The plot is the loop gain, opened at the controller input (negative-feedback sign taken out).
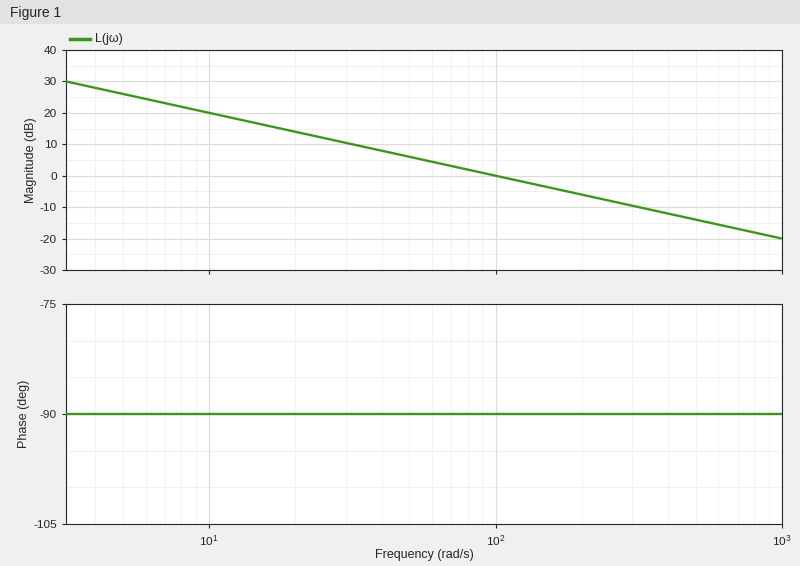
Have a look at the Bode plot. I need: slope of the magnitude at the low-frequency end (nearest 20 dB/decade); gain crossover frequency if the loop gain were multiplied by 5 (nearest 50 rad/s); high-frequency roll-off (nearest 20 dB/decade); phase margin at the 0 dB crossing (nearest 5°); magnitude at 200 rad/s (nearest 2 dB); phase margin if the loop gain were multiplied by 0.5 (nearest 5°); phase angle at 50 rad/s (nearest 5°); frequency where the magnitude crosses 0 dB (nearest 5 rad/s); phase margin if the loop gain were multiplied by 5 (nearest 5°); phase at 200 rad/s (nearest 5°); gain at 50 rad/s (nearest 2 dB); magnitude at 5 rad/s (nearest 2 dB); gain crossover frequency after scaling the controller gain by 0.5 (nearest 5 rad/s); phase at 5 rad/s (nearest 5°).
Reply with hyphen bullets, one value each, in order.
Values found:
- -20 dB/decade
- 500 rad/s
- -20 dB/decade
- 90°
- -6 dB
- 90°
- -90°
- 100 rad/s
- 90°
- -90°
- 6 dB
- 26 dB
- 50 rad/s
- -90°
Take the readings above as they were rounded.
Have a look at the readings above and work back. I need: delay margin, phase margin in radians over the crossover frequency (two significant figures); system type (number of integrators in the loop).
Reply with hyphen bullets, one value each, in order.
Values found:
- 0.016 s
- 1
